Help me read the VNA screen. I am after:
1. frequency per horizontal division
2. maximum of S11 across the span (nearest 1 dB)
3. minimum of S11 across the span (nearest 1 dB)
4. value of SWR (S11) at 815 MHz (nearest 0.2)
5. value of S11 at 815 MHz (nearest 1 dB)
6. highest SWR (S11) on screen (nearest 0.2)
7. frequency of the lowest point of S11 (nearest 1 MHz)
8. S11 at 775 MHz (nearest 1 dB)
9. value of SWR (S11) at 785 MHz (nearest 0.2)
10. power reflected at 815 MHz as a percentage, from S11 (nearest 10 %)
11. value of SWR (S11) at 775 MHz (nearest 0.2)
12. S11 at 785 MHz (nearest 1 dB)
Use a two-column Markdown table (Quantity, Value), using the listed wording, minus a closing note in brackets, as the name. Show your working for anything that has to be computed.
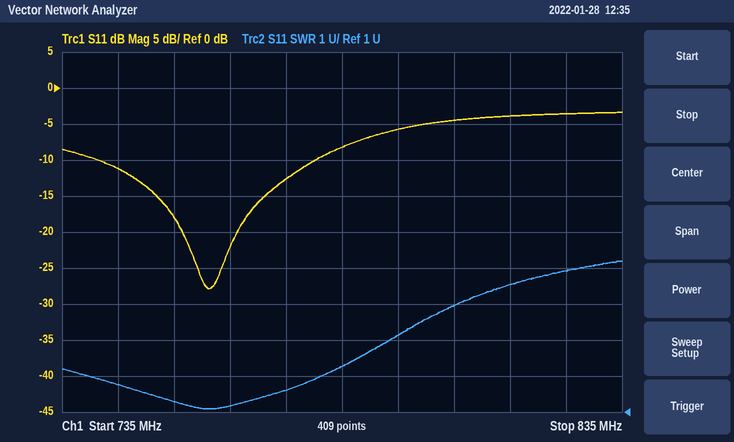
| Quantity | Value |
|---|---|
| frequency per horizontal division | 10 MHz |
| maximum of S11 across the span | -3 dB |
| minimum of S11 across the span | -28 dB |
| value of SWR (S11) at 815 MHz | 4.6 |
| value of S11 at 815 MHz | -4 dB |
| highest SWR (S11) on screen | 5.2 |
| frequency of the lowest point of S11 | 761 MHz |
| S11 at 775 MHz | -13 dB |
| value of SWR (S11) at 785 MHz | 2.2 |
| power reflected at 815 MHz as a percentage, from S11 | 10^(-4/10) ≈ 40 % |
| value of SWR (S11) at 775 MHz | 1.6 |
| S11 at 785 MHz | -8 dB |
